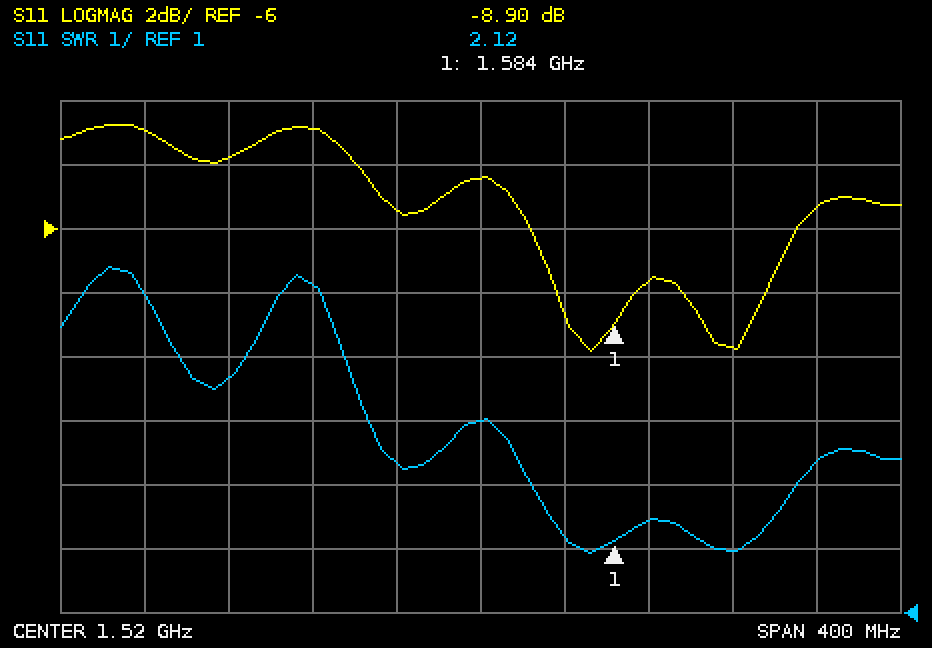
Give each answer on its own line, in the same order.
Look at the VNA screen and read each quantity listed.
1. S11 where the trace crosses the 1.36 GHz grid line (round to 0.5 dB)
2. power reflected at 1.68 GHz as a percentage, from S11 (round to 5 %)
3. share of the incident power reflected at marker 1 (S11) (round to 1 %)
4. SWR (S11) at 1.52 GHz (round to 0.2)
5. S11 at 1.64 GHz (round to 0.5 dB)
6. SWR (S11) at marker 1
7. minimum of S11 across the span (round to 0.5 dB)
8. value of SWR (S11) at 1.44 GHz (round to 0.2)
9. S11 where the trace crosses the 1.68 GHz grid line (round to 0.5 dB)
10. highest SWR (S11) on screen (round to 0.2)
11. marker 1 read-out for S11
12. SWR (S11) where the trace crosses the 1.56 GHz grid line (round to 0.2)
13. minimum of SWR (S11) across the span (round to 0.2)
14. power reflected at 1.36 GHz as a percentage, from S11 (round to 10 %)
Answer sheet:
-3.0 dB
30 %
13 %
4.0
-9.5 dB
2.12
-10.0 dB
6.2
-5.5 dB
6.4
-8.90 dB
2.2
2.0
50 %
